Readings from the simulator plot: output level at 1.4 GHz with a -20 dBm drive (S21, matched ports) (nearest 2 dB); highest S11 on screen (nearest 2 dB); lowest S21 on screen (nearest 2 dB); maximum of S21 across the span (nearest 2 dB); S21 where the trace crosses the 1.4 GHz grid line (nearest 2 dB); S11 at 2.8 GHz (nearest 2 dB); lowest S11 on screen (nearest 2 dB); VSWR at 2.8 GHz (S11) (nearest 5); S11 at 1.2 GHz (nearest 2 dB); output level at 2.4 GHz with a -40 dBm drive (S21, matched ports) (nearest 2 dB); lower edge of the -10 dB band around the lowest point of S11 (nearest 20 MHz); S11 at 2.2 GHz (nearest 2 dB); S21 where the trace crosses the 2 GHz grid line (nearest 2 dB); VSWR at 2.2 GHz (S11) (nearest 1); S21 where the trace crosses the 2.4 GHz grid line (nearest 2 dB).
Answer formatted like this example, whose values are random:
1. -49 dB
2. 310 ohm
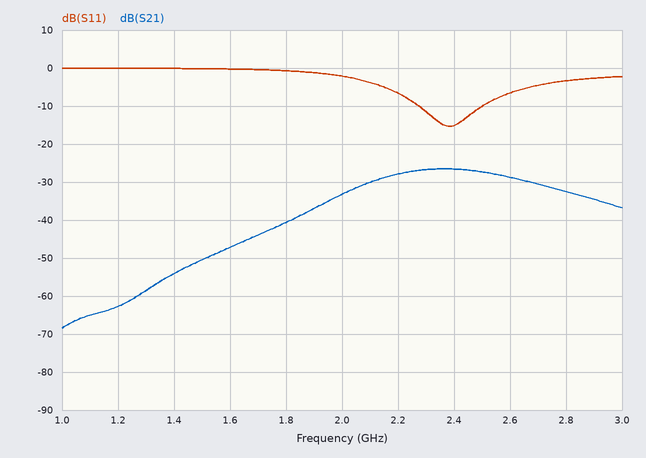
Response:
1. -74 dBm
2. 0 dB
3. -68 dB
4. -26 dB
5. -54 dB
6. -4 dB
7. -16 dB
8. 5
9. 0 dB
10. -66 dBm
11. 2.28 GHz
12. -6 dB
13. -34 dB
14. 3
15. -26 dB
